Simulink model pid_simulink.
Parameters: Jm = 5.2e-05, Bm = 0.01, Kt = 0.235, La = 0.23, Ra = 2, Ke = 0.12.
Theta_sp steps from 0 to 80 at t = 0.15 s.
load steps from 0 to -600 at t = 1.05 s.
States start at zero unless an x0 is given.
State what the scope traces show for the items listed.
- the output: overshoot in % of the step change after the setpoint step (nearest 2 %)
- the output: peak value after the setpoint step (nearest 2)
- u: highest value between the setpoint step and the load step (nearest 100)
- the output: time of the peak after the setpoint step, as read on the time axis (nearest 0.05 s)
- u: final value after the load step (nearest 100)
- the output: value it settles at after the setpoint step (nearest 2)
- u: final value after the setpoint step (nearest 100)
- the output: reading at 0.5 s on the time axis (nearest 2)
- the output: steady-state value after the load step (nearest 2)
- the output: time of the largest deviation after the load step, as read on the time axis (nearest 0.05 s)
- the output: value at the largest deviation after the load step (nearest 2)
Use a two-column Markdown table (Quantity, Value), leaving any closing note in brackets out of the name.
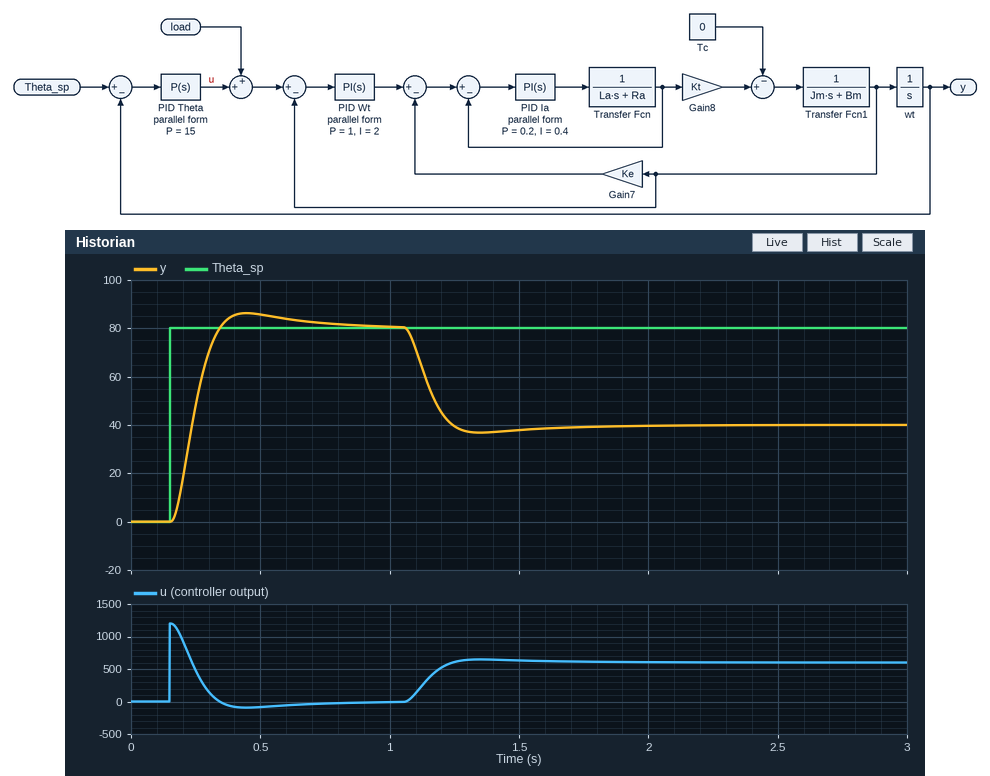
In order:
| Quantity | Value |
|---|---|
| the output: overshoot in % of the step change after the setpoint step | 8 % |
| the output: peak value after the setpoint step | 86 |
| u: highest value between the setpoint step and the load step | 1200 |
| the output: time of the peak after the setpoint step, as read on the time axis | 0.45 s |
| u: final value after the load step | 600 |
| the output: value it settles at after the setpoint step | 80 |
| u: final value after the setpoint step | 0 |
| the output: reading at 0.5 s on the time axis | 86 |
| the output: steady-state value after the load step | 40 |
| the output: time of the largest deviation after the load step, as read on the time axis | 1.35 s |
| the output: value at the largest deviation after the load step | 36 |
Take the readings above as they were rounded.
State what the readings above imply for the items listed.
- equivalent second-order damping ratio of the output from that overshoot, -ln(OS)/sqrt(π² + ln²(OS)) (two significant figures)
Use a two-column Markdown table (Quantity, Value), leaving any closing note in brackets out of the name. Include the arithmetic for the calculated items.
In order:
| Quantity | Value |
|---|---|
| equivalent second-order damping ratio of the output from that overshoot, -ln(OS)/sqrt(π² + ln²(OS)) | ln(0.08) = -2.526; 2.526 / sqrt(9.870 + 6.379) = 0.63 |
